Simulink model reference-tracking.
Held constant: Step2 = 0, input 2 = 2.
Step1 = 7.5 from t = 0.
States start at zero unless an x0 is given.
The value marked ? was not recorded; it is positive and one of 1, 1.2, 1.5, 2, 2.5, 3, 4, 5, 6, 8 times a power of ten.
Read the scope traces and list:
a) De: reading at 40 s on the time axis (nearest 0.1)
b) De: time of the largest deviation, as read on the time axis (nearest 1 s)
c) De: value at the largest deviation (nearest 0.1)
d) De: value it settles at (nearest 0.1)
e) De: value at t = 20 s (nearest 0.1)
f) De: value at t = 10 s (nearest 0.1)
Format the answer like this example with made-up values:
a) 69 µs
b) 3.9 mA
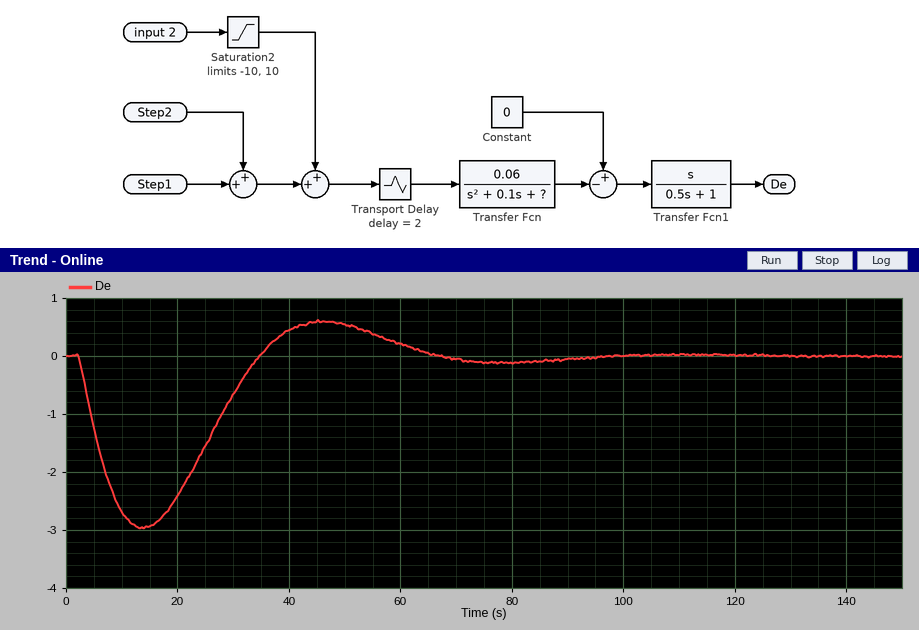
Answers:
a) 0.4
b) 14 s
c) -3.0
d) 0.0
e) -2.4
f) -2.7
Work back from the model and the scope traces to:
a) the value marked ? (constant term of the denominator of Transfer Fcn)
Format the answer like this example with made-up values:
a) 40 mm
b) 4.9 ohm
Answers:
a) 0.012
